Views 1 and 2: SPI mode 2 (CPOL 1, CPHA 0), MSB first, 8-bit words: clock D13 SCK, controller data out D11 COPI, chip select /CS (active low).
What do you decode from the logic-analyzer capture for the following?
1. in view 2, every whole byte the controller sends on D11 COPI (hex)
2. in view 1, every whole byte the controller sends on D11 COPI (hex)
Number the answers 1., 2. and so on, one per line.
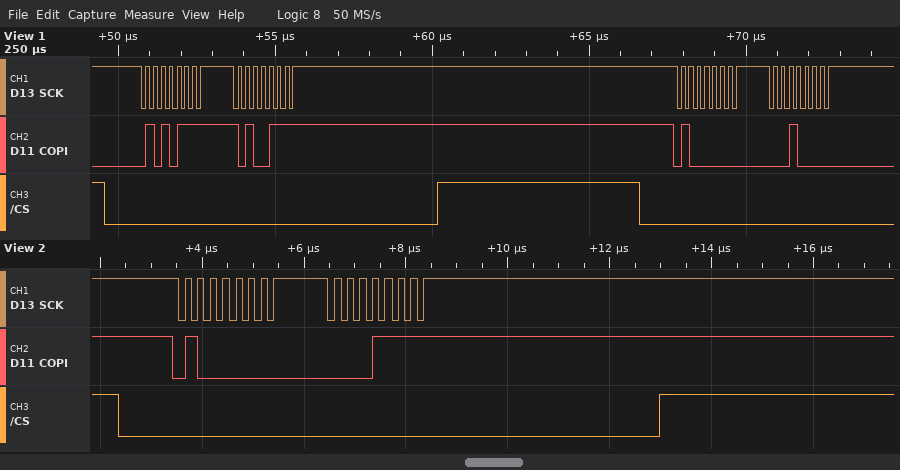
1. 40 0F
2. 0x57 0xA7 0x40 0x10
